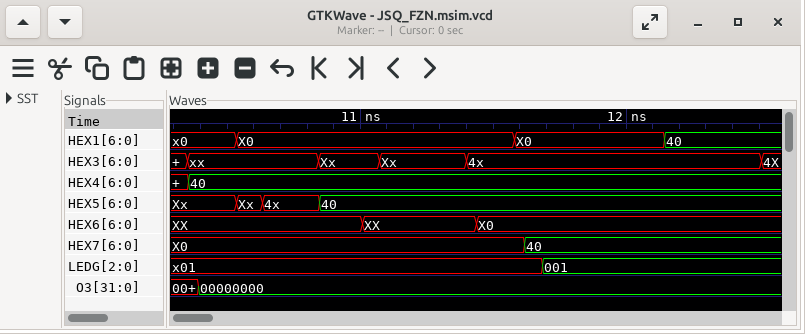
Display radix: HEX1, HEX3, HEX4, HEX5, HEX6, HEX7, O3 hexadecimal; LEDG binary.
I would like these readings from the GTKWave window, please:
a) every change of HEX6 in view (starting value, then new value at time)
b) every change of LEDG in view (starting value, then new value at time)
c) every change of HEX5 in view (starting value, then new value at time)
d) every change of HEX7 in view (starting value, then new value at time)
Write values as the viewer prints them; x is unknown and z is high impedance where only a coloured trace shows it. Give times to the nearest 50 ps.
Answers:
XX, XX at 11000 ps, X0 at 11450 ps
x01, 001 at 11700 ps
Xx, Xx at 10550 ps, 4x at 10650 ps, 40 at 10850 ps
X0, 40 at 11600 ps
